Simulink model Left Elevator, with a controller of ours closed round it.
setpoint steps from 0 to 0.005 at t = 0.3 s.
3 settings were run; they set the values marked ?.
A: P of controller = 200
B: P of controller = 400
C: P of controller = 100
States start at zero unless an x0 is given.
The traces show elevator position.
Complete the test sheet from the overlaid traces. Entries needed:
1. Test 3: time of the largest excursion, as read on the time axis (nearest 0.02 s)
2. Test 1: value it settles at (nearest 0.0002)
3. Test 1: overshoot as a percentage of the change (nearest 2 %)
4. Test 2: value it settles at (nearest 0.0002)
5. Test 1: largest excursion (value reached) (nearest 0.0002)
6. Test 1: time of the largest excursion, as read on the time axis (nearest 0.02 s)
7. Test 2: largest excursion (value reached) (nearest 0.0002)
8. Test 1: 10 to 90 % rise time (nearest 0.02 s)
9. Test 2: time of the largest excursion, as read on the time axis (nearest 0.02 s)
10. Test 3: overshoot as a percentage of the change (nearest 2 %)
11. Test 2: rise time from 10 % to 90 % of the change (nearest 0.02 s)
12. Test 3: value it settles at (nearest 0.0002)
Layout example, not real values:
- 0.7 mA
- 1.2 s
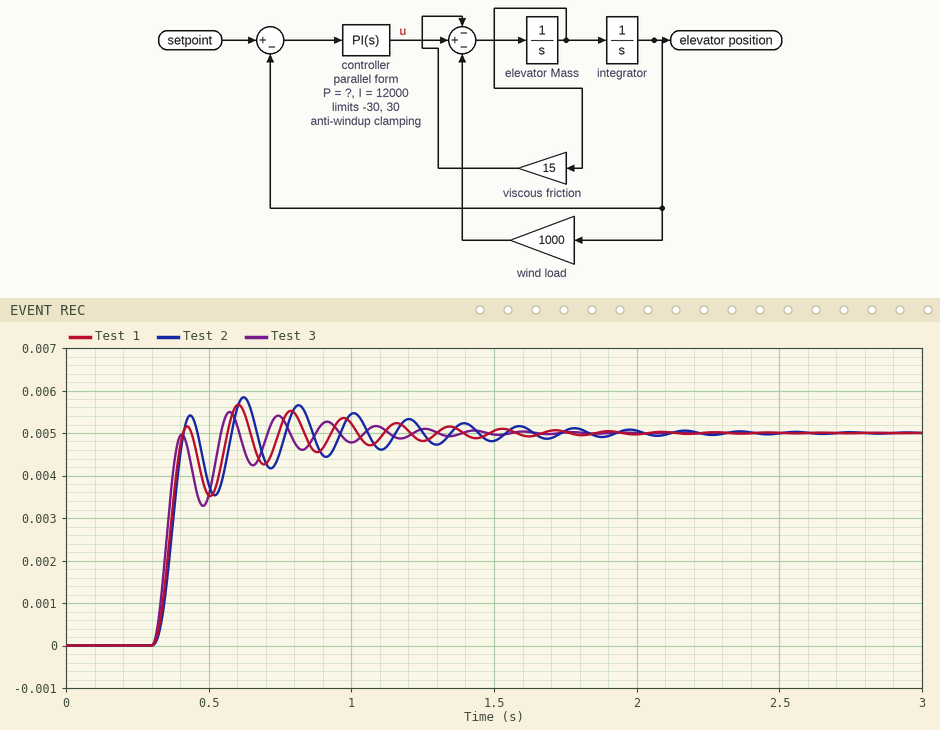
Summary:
- 0.58 s
- 0.0050
- 14 %
- 0.0050
- 0.0056
- 0.60 s
- 0.0058
- 0.06 s
- 0.62 s
- 10 %
- 0.06 s
- 0.0050
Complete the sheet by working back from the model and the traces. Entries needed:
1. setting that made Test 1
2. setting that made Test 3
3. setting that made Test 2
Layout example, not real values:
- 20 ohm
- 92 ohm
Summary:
- A
- B
- C
